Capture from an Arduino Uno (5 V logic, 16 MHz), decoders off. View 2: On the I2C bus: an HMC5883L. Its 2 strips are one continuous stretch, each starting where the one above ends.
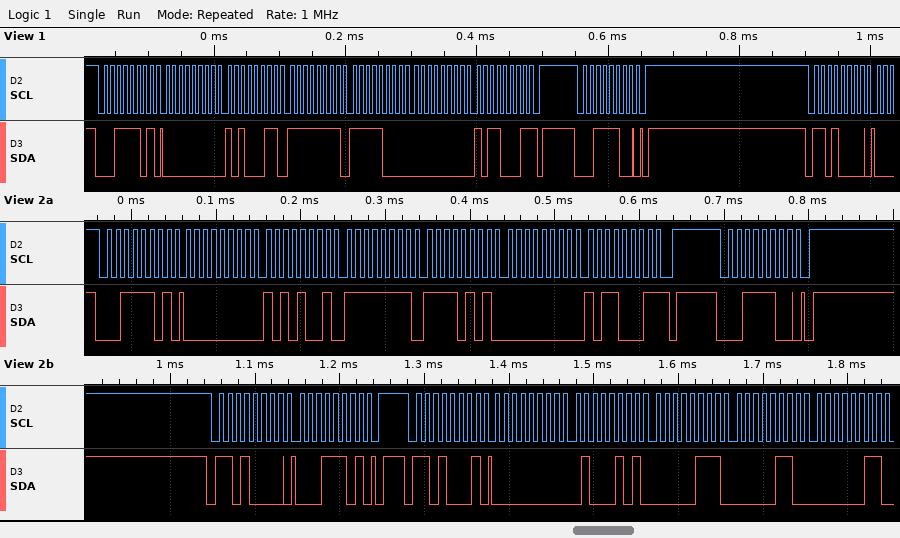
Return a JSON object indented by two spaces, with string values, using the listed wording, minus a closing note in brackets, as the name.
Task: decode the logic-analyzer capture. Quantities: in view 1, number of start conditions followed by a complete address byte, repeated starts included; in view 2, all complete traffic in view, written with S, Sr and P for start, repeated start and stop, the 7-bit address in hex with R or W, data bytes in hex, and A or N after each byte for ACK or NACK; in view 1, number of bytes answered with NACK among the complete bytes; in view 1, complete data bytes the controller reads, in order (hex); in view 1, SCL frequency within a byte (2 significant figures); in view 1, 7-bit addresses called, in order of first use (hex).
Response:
{
  "in view 1, number of start conditions followed by a complete address byte, repeated starts included": "3",
  "in view 2, all complete traffic in view, written with S, Sr and P for start, repeated start and stop, the 7-bit address in hex with R or W, data bytes in hex, and A or N after each byte for ACK or NACK": "S 1ER A 00 A A9 A FF A F5 A 00 A B1 N P S 1EW A P S 68W A 1D A P S 68R A 00 A 45 A 07 A 06 A 03 A",
  "in view 1, number of bytes answered with NACK among the complete bytes": "1",
  "in view 1, complete data bytes the controller reads, in order": "00 A3 FF F8 00 B1",
  "in view 1, SCL frequency within a byte": "100 kHz",
  "in view 1, 7-bit addresses called, in order of first use": "0x1E 0x68"
}
